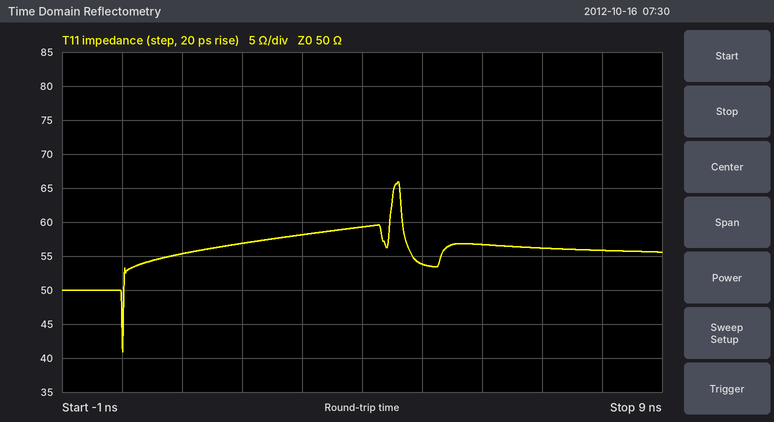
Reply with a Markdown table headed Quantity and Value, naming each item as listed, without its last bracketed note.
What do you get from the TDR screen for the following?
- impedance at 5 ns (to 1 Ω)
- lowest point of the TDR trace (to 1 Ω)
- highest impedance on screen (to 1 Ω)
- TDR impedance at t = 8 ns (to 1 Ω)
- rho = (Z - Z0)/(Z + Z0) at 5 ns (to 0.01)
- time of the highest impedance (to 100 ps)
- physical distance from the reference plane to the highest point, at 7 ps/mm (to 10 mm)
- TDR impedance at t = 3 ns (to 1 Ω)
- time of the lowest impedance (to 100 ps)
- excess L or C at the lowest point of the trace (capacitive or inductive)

| Quantity | Value |
|---|---|
| impedance at 5 ns | 54 Ω |
| lowest point of the TDR trace | 41 Ω |
| highest impedance on screen | 66 Ω |
| TDR impedance at t = 8 ns | 56 Ω |
| rho = (Z - Z0)/(Z + Z0) at 5 ns | +0.04 |
| time of the highest impedance | 4.6 ns |
| physical distance from the reference plane to the highest point, at 7 ps/mm | 330 mm |
| TDR impedance at t = 3 ns | 58 Ω |
| time of the lowest impedance | 0.0 ns |
| excess L or C at the lowest point of the trace | capacitive |
